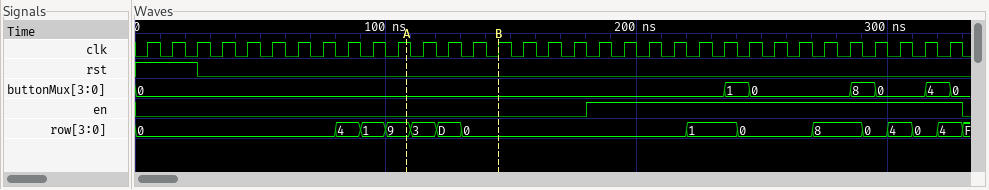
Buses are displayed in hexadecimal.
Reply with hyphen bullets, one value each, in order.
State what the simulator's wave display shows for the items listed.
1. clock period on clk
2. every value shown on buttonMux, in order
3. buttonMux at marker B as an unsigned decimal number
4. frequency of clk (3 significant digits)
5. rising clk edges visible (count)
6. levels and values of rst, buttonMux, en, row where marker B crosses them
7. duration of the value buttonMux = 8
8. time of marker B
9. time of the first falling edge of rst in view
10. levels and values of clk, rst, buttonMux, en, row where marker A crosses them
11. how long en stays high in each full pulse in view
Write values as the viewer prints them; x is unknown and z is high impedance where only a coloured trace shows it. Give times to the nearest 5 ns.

- 10 ns
- 0, 1, 0, 8, 0, 4, 0
- 0
- 100 MHz
- 33
- rst=0, buttonMux=0, en=0, row=0
- 10 ns
- 145 ns
- 25 ns
- clk=1, rst=0, buttonMux=0, en=0, row=9
- 150 ns
